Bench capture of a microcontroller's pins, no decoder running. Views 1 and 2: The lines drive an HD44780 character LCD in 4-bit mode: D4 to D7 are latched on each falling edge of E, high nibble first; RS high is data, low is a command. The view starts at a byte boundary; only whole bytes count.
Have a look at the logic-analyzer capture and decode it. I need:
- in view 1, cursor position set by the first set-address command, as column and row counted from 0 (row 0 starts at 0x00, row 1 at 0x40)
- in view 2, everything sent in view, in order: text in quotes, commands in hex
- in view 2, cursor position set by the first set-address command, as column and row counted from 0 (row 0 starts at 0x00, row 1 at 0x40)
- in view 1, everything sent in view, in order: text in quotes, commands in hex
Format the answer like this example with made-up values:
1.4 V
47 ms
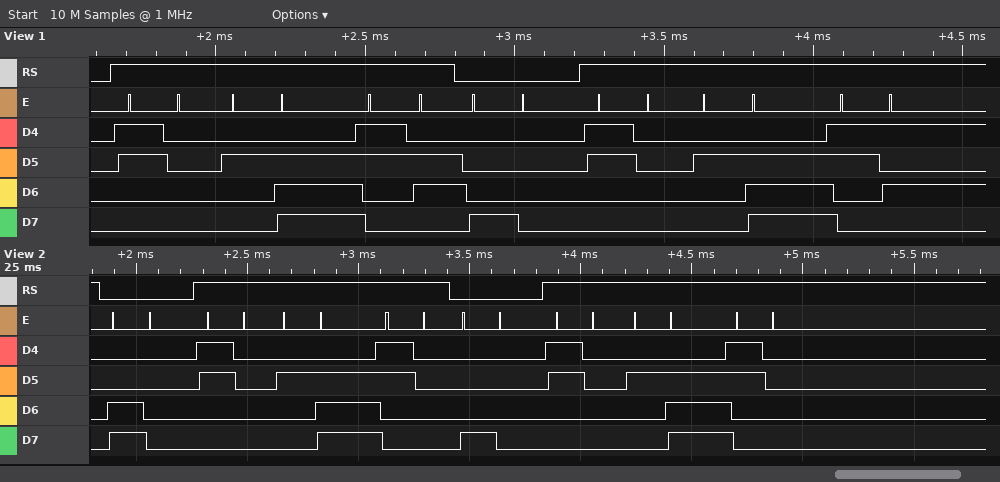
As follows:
column 0, row 0
0xC0 "0.0" 0x80 "0.0"
column 0, row 1
"0.6" 0x80 "0.5"
